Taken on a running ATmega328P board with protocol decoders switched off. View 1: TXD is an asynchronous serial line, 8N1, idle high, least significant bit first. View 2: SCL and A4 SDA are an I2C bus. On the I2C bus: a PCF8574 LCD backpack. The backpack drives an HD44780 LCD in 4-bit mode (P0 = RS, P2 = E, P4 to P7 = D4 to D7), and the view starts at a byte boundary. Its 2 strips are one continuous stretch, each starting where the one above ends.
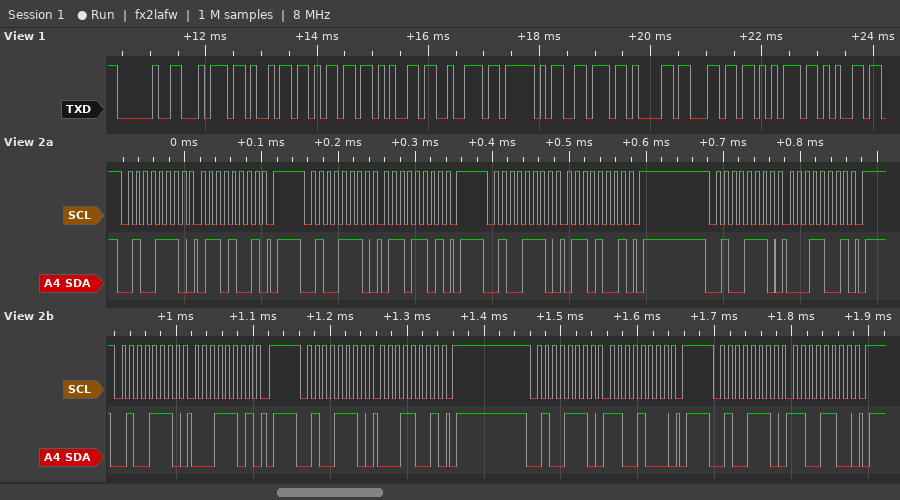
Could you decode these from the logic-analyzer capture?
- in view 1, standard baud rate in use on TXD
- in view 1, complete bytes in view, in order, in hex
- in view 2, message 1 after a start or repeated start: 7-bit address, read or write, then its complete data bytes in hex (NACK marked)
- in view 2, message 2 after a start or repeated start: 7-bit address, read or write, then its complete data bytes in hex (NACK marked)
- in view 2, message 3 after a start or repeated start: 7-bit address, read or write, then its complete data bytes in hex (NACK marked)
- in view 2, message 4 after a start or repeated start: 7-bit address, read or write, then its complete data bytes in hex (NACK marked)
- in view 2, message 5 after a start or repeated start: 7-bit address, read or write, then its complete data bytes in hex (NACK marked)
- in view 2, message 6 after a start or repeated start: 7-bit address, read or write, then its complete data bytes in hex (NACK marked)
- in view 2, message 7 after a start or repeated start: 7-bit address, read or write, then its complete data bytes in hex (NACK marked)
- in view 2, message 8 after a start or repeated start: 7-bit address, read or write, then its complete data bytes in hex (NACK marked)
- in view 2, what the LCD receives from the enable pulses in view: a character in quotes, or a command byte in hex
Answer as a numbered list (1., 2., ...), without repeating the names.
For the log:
1. 9600 baud
2. 20 74 69 6D 65 72 5F 76 61 6C 75 65
3. 0x27 write: 69
4. 0x27 write: 6D
5. 0x27 write: 69
6. 0x27 write: 19
7. 0x27 write: 1D
8. 0x27 write: 19
9. 0x27 write: C8
10. 0x27 write: CC
11. 'a'
